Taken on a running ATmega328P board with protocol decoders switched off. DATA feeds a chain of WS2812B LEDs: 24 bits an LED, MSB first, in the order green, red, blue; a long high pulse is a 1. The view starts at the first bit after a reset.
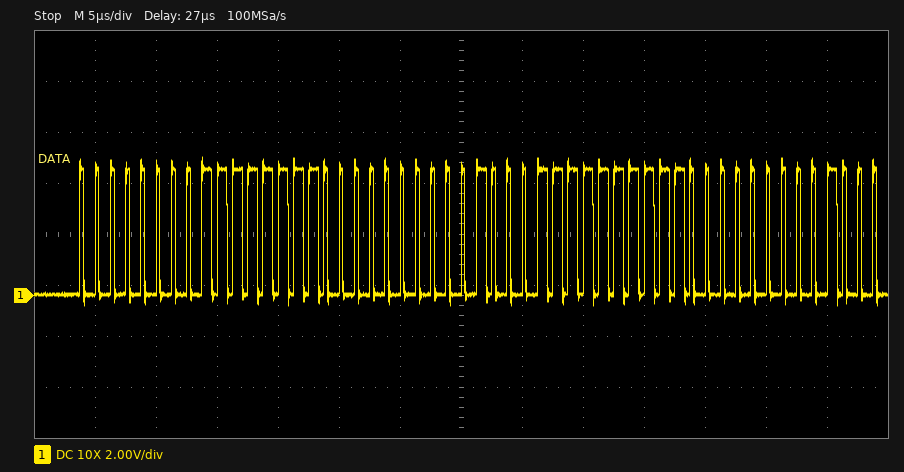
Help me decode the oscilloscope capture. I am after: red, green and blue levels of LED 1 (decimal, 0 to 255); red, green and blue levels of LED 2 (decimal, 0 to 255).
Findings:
255, 0, 0
255, 35, 0
